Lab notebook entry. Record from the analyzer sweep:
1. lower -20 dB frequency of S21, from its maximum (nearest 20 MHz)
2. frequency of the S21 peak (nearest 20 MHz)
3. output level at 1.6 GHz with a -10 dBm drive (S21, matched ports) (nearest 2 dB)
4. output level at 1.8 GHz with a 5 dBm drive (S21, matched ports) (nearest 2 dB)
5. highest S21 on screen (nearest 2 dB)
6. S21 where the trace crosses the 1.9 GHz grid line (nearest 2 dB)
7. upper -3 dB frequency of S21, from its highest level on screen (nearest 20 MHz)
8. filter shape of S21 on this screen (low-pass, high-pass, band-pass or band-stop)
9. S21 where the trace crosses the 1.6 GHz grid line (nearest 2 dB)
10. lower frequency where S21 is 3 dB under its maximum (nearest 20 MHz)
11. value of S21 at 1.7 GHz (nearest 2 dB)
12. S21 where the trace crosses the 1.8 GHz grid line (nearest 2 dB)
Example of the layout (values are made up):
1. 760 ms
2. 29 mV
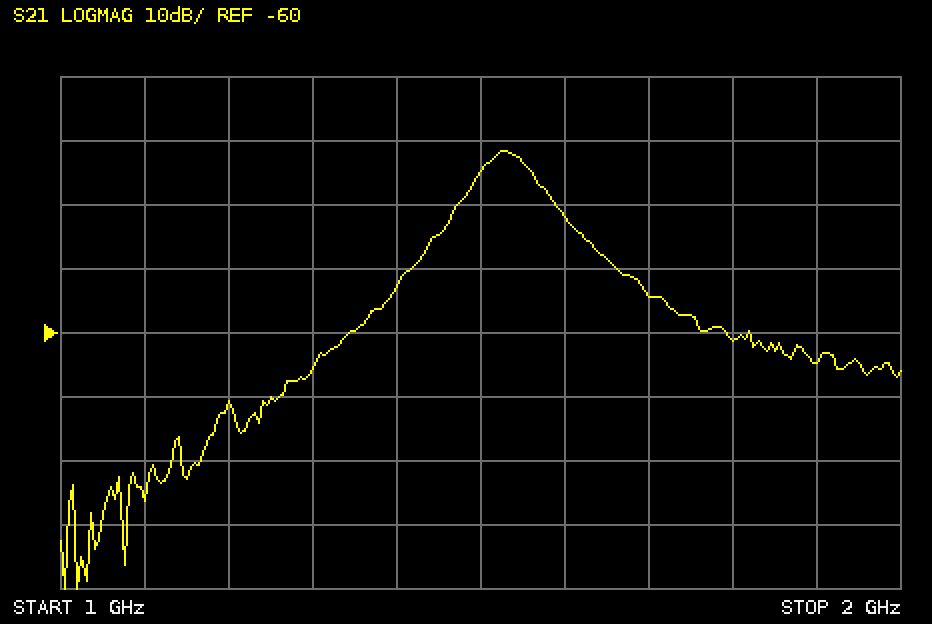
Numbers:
1. 1.40 GHz
2. 1.52 GHz
3. -52 dBm
4. -56 dBm
5. -32 dB
6. -64 dB
7. 1.56 GHz
8. band-pass
9. -42 dB
10. 1.50 GHz
11. -54 dB
12. -62 dB
